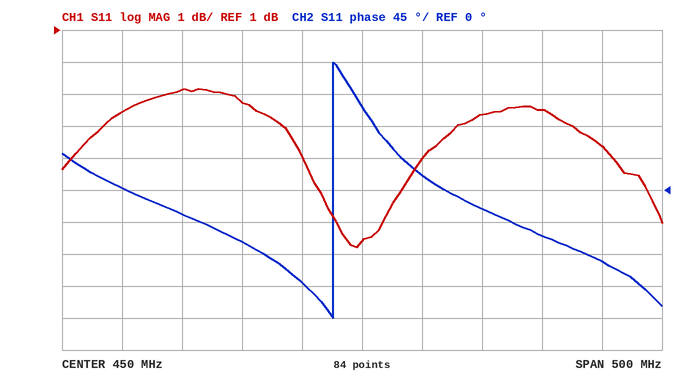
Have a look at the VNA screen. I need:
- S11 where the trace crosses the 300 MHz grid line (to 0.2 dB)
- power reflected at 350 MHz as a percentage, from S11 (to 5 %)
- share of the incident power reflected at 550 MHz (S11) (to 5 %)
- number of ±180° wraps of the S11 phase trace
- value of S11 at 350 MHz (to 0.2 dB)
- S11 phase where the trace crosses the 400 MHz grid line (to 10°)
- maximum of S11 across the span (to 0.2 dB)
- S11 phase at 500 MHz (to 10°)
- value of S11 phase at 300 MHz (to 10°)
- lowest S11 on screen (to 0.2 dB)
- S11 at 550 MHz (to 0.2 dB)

-0.8 dB
75 %
70 %
1
-1.2 dB
-130°
-0.8 dB
20°
-30°
-5.8 dB
-1.6 dB
